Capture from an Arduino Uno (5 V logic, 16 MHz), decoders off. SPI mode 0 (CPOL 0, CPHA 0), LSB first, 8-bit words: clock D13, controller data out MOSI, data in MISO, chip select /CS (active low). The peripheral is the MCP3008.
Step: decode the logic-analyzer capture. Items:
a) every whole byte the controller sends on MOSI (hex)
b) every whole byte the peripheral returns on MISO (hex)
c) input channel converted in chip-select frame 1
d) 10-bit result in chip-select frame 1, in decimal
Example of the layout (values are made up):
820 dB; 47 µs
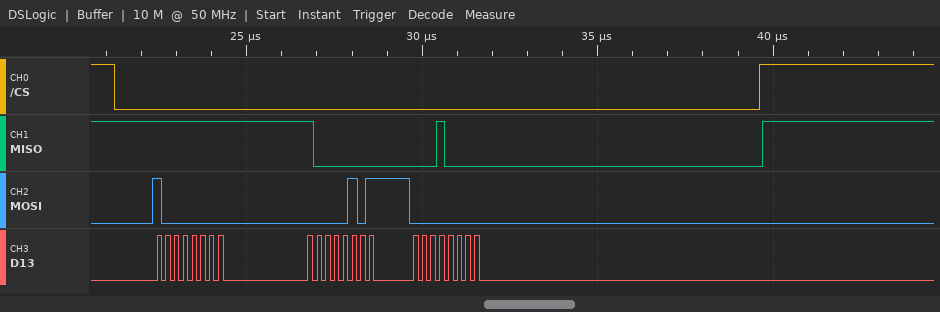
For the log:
01 A0 00; FF 01 08; 2; 264
